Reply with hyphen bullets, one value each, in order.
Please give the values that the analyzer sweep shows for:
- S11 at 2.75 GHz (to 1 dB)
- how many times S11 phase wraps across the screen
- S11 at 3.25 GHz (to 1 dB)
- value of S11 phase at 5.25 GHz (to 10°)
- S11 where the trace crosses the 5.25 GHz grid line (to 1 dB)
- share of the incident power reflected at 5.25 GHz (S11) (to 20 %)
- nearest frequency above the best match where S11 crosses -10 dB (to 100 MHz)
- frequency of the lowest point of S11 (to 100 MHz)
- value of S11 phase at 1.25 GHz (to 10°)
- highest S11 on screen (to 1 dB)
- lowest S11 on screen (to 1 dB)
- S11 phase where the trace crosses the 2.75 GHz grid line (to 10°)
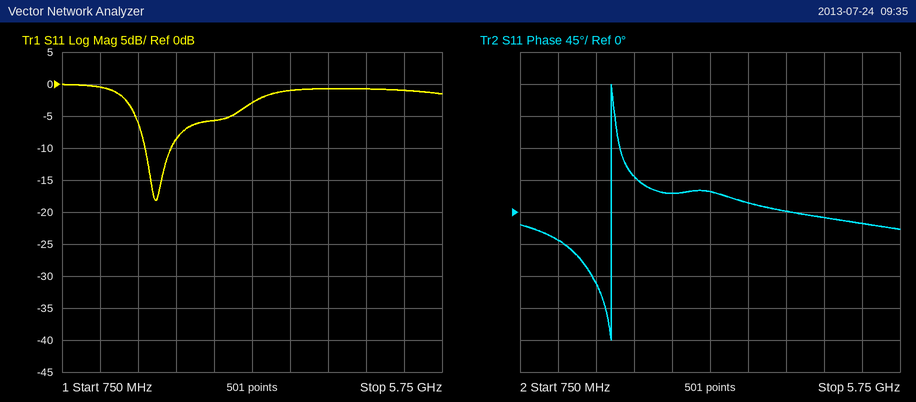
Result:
- -6 dB
- 1
- -3 dB
- -20°
- -1 dB
- 80 %
- 2.2 GHz
- 2.0 GHz
- -40°
- 0 dB
- -18 dB
- 30°
